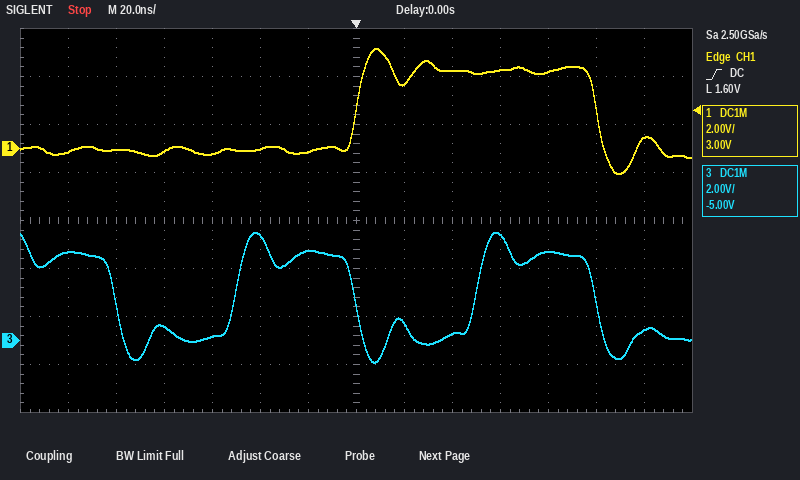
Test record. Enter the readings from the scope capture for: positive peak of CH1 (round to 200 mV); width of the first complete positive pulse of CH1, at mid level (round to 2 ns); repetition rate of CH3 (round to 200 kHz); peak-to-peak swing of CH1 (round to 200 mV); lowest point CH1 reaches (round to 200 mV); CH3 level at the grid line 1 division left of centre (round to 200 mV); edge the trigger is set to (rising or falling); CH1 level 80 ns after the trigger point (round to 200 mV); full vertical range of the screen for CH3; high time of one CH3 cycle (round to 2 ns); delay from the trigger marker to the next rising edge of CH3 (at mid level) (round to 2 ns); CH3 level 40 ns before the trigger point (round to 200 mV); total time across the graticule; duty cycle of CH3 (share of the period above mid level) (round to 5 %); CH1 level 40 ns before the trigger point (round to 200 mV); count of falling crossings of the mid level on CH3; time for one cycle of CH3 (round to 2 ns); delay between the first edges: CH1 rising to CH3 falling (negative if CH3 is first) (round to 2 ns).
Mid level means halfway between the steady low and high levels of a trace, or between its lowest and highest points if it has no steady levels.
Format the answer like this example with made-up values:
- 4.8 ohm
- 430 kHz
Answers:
- 4.2 V
- 100 ns
- 10.0 MHz
- 5.2 V
- -1.0 V
- 3.8 V
- rising
- 3.2 V
- 16 V
- 50 ns
- 50 ns
- 4.4 V
- 280 ns
- 50 %
- 0.0 V
- 3
- 100 ns
- -100 ns
